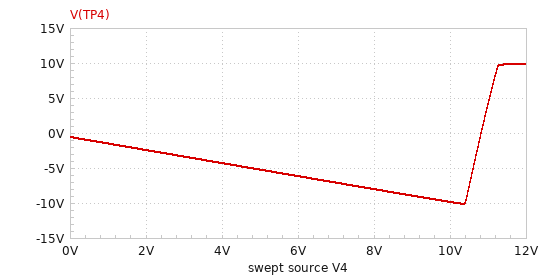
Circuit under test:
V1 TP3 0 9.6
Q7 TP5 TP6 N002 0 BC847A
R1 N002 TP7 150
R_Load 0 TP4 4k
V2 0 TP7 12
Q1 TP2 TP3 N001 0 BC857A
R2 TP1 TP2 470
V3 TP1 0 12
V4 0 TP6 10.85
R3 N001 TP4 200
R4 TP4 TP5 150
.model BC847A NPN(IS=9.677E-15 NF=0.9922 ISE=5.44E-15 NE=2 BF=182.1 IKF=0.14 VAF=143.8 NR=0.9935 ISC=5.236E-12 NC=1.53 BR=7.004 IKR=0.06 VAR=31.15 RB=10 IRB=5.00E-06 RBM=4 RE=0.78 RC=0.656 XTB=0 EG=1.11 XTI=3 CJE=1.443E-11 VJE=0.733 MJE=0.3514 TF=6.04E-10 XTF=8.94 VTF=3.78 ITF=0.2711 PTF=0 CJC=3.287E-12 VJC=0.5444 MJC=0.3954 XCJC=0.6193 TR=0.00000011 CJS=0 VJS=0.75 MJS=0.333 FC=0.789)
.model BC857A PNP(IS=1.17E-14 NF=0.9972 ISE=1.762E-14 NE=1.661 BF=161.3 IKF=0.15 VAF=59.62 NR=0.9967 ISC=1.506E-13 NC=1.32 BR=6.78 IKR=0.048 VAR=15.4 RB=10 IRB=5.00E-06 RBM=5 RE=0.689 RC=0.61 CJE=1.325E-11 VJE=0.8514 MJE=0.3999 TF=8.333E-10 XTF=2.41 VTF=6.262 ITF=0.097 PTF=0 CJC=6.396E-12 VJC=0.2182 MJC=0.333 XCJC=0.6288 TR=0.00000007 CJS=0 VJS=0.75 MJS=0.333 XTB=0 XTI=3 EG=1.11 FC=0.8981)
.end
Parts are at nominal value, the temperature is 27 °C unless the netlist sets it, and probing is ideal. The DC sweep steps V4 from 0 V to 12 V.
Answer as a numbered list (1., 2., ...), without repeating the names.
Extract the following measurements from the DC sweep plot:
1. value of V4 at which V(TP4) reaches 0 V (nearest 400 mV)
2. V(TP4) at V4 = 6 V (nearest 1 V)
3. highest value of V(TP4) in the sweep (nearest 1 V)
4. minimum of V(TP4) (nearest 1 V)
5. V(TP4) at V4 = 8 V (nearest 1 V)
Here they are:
1. 10.8 V
2. -6 V
3. 10 V
4. -10 V
5. -8 V
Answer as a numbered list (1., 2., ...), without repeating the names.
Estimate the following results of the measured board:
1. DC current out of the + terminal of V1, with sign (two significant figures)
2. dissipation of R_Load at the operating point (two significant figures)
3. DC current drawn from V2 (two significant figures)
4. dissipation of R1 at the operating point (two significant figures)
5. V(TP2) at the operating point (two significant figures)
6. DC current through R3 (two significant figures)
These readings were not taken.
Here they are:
1. -380 µA
2. 130 µW
3. 3.1 mA
4. 1.5 mW
5. 10 V
6. 3.3 mA
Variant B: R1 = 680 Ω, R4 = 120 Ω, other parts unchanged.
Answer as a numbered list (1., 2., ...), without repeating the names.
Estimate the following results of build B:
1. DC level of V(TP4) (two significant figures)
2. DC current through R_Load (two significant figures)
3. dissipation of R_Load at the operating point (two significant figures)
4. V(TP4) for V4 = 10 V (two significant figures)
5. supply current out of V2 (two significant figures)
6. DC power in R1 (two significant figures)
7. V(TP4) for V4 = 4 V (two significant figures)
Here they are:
1. 9.3 V
2. 2.3 mA
3. 22 mW
4. 5.0 V
5. 750 µA
6. 380 µW
7. -4.2 V
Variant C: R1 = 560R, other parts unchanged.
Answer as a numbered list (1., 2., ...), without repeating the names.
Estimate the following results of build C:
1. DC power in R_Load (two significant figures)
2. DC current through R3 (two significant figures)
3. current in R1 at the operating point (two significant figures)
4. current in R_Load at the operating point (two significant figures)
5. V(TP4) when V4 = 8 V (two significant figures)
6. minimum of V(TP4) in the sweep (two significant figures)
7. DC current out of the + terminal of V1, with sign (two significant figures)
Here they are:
1. 19 mW
2. 3.1 mA
3. 900 µA
4. 2.2 mA
5. -7.9 V
6. -8.0 V
7. -550 µA
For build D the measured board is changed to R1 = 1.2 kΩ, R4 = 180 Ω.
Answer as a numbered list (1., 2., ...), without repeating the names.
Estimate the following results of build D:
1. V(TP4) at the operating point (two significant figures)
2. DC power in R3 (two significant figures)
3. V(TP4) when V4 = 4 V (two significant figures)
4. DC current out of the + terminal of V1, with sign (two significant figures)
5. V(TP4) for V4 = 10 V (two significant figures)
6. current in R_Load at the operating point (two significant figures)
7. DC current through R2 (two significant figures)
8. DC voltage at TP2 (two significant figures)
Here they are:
1. 9.7 V
2. 1.6 mW
3. -3.9 V
4. -770 µA
5. 8.0 V
6. 2.4 mA
7. 3.6 mA
8. 10 V
